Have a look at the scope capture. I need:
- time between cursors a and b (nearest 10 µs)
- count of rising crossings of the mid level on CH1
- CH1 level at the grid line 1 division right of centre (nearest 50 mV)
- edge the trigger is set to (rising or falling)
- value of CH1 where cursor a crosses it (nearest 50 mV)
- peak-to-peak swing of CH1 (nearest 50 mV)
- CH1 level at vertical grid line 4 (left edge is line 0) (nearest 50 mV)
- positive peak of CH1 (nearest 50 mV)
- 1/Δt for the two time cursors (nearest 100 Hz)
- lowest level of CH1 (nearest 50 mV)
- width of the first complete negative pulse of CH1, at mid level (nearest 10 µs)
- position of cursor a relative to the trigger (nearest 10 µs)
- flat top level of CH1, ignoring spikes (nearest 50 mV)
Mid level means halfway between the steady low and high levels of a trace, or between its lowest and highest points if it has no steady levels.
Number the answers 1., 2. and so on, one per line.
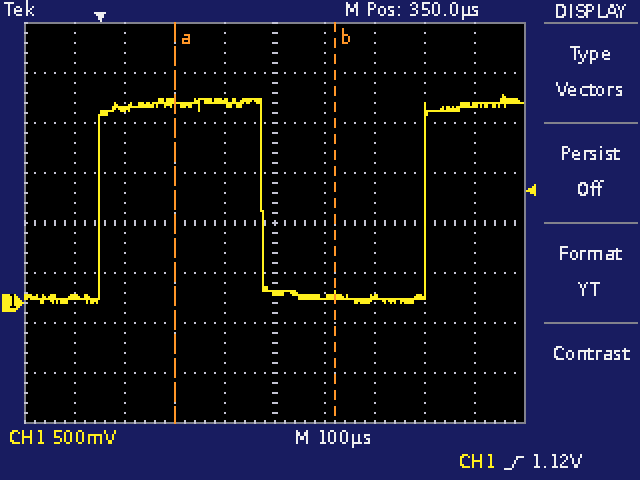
1. 320 µs
2. 2
3. 50 mV
4. rising
5. 2.00 V
6. 2.10 V
7. 2.00 V
8. 2.10 V
9. 3.1 kHz
10. 0 mV
11. 330 µs
12. +150 µs
13. 2.00 V
